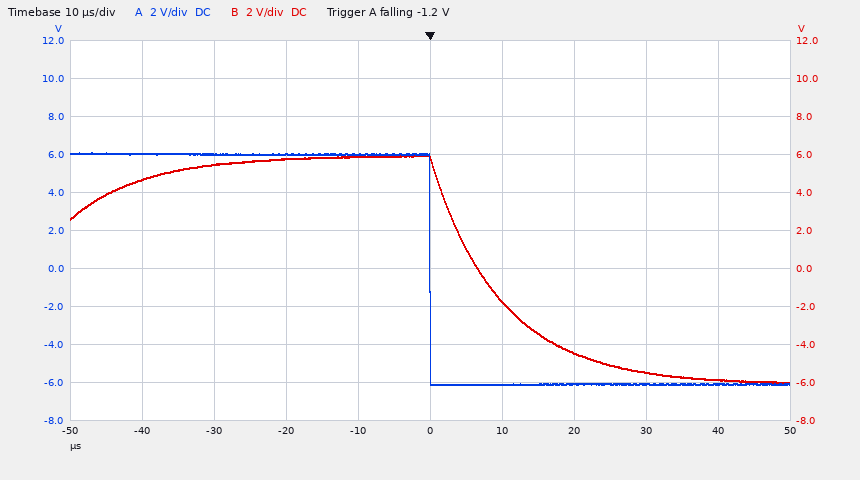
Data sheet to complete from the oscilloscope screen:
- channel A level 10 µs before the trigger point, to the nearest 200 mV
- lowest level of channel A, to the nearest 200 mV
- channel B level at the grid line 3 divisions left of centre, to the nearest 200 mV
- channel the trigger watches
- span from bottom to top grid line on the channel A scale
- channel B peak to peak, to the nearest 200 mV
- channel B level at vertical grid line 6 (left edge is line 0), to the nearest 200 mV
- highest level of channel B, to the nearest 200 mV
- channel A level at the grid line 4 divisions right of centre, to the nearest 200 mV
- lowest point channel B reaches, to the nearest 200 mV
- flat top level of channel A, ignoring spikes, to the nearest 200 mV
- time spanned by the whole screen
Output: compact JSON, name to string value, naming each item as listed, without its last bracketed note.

{"channel A level 10 µs before the trigger point, to the nearest 200 mV": "6.0 V", "lowest level of channel A, to the nearest 200 mV": "-6.2 V", "channel B level at the grid line 3 divisions left of centre, to the nearest 200 mV": "5.4 V", "channel the trigger watches": "channel A", "span from bottom to top grid line on the channel A scale": "20 V", "channel B peak to peak, to the nearest 200 mV": "12.0 V", "channel B level at vertical grid line 6 (left edge is line 0), to the nearest 200 mV": "-1.8 V", "highest level of channel B, to the nearest 200 mV": "6.0 V", "channel A level at the grid line 4 divisions right of centre, to the nearest 200 mV": "-6.0 V", "lowest point channel B reaches, to the nearest 200 mV": "-6.0 V", "flat top level of channel A, ignoring spikes, to the nearest 200 mV": "6.0 V", "time spanned by the whole screen": "100 µs"}
